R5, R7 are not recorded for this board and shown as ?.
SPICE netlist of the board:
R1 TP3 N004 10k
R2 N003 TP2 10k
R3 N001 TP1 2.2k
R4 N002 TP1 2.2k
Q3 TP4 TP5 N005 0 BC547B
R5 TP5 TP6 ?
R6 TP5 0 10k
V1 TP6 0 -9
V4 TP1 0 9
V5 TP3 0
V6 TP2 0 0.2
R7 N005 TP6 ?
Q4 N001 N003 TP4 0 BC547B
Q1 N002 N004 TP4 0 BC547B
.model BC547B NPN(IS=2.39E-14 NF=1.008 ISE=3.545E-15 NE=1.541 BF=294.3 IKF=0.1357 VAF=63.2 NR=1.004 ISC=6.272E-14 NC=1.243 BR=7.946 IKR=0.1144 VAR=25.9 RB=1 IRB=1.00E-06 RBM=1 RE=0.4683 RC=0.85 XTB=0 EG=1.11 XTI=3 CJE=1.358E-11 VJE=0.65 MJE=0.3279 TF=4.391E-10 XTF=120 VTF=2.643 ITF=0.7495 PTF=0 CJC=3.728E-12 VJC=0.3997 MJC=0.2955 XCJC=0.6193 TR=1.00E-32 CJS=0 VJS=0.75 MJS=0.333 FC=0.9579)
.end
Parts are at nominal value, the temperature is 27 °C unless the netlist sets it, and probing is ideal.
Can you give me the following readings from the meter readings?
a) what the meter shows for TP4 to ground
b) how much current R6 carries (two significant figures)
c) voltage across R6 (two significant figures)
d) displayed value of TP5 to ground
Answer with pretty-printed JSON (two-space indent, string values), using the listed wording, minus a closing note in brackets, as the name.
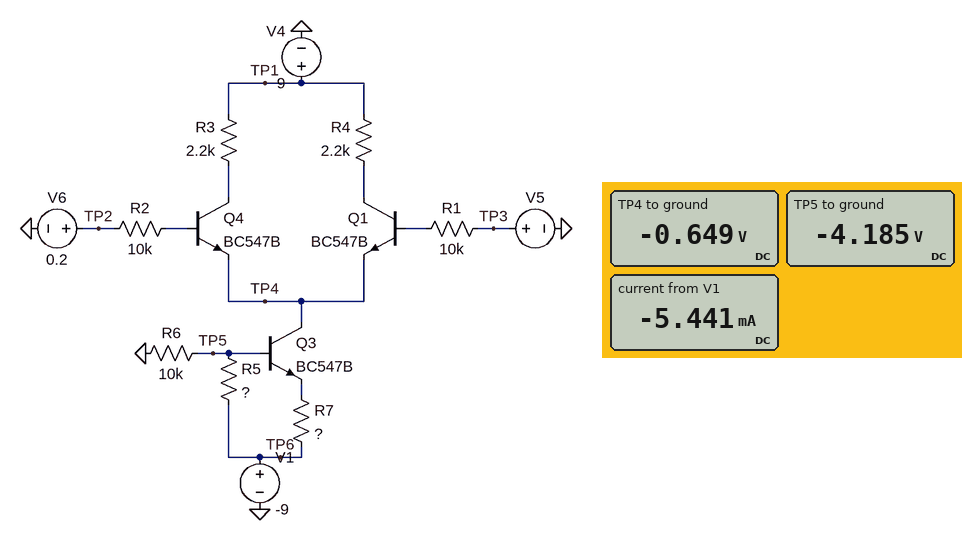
{
  "what the meter shows for TP4 to ground": "-0.649 V",
  "how much current R6 carries": "420 µA",
  "voltage across R6": "4.2 V",
  "displayed value of TP5 to ground": "-4.185 V"
}
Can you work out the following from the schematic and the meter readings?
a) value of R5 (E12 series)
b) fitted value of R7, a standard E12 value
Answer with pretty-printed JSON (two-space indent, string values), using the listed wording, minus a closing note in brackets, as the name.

{
  "value of R5": "12 kΩ",
  "fitted value of R7, a standard E12 value": "820 Ω"
}
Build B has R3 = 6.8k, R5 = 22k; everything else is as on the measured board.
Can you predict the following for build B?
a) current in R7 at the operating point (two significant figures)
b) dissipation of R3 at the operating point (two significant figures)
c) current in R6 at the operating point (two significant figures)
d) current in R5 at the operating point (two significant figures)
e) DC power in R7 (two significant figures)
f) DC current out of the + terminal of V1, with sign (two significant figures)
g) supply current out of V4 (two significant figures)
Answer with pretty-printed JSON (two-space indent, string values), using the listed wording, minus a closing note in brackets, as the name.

{
  "current in R7 at the operating point": "6.5 mA",
  "dissipation of R3 at the operating point": "16 mW",
  "current in R6 at the operating point": "300 µA",
  "current in R5 at the operating point": "270 µA",
  "DC power in R7": "35 mW",
  "DC current out of the + terminal of V1, with sign": "-6.8 mA",
  "supply current out of V4": "6.3 mA"
}
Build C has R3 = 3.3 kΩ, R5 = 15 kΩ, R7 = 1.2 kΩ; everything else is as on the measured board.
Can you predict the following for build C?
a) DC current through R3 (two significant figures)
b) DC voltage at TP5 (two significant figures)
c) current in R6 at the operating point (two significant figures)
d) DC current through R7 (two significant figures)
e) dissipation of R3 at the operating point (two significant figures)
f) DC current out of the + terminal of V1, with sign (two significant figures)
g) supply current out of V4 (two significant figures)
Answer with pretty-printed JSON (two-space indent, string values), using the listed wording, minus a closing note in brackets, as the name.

{
  "DC current through R3": "2.9 mA",
  "DC voltage at TP5": "-3.7 V",
  "current in R6 at the operating point": "370 µA",
  "DC current through R7": "3.9 mA",
  "dissipation of R3 at the operating point": "28 mW",
  "DC current out of the + terminal of V1, with sign": "-4.2 mA",
  "supply current out of V4": "3.8 mA"
}
